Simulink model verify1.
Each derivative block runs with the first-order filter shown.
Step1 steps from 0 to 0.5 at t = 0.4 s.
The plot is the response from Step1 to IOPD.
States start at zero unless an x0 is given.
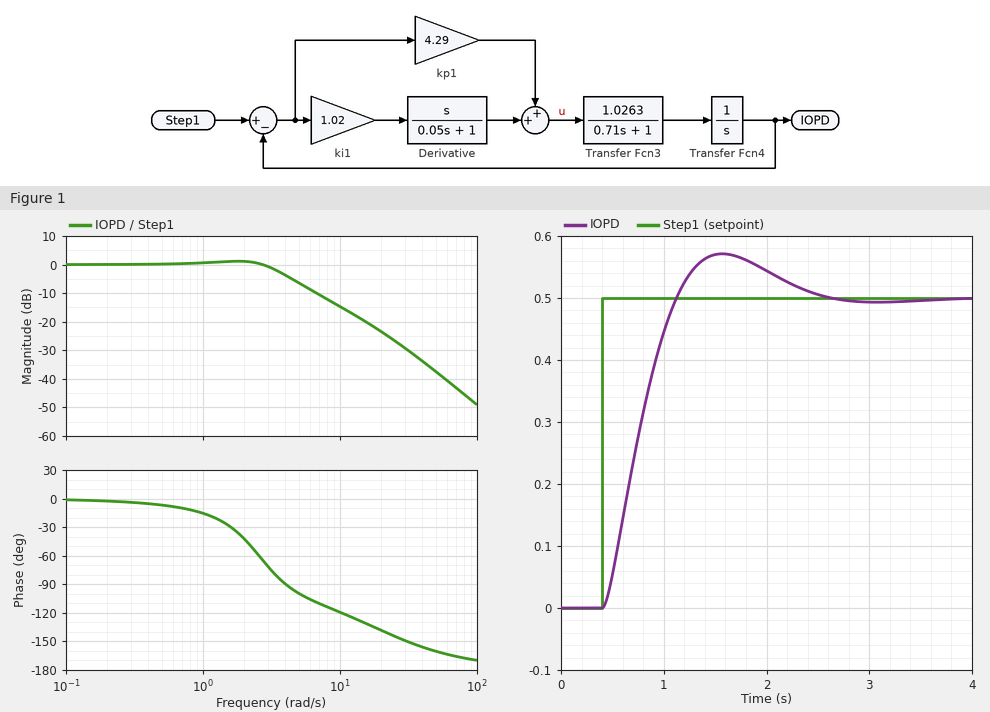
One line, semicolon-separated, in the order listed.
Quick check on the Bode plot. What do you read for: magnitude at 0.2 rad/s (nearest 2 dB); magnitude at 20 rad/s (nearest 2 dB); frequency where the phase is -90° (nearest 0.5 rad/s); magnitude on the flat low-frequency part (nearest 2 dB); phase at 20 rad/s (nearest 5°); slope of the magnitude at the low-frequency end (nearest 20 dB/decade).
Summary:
0 dB; -24 dB; 4.0 rad/s; 0 dB; -140°; 0 dB/decade
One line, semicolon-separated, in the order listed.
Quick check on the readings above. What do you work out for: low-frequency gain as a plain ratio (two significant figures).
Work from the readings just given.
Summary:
1.0
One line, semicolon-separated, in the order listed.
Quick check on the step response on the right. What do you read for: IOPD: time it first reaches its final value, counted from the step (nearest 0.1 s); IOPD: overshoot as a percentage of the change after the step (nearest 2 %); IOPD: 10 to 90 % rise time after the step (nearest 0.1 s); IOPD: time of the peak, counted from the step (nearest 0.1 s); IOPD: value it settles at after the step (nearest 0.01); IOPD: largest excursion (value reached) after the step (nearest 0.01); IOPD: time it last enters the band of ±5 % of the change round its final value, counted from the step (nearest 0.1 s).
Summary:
0.7 s; 14 %; 0.5 s; 1.2 s; 0.50; 0.57; 1.8 s
